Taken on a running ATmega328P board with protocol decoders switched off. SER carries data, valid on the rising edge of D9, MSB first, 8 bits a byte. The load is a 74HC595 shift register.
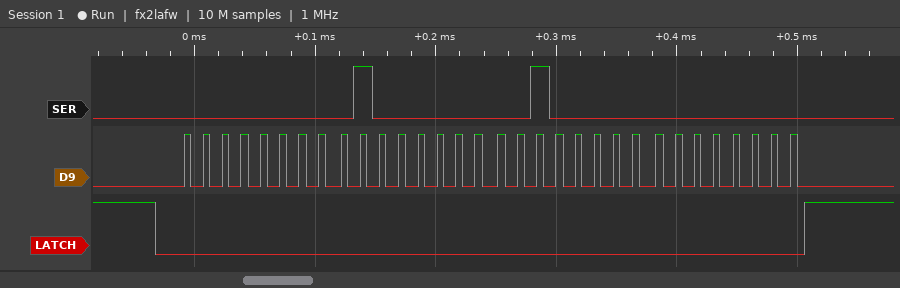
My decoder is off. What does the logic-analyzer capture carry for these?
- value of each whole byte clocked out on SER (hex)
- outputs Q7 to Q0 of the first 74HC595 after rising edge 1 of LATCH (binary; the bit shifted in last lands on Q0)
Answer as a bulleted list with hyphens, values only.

- 00 40 20 00
- 00000000
